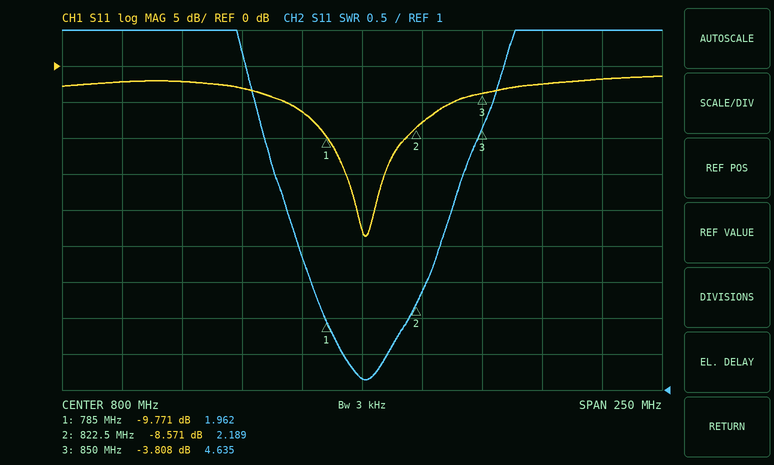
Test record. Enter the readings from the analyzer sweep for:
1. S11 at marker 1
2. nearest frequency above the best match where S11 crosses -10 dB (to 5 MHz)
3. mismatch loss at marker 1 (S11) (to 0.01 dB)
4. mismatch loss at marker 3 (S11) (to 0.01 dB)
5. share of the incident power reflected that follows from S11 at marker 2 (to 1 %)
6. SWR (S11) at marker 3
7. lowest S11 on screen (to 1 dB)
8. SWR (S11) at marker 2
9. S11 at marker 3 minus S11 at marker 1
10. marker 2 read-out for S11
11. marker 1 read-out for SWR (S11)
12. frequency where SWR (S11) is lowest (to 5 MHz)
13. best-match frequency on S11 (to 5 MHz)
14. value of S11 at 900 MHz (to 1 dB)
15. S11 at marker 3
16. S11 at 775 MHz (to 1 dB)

-9.771 dB
820 MHz
0.48 dB
2.34 dB
14 %
4.635
-24 dB
2.189
5.963 dB
-8.571 dB
1.962
800 MHz
800 MHz
-2 dB
-3.808 dB
-6 dB
